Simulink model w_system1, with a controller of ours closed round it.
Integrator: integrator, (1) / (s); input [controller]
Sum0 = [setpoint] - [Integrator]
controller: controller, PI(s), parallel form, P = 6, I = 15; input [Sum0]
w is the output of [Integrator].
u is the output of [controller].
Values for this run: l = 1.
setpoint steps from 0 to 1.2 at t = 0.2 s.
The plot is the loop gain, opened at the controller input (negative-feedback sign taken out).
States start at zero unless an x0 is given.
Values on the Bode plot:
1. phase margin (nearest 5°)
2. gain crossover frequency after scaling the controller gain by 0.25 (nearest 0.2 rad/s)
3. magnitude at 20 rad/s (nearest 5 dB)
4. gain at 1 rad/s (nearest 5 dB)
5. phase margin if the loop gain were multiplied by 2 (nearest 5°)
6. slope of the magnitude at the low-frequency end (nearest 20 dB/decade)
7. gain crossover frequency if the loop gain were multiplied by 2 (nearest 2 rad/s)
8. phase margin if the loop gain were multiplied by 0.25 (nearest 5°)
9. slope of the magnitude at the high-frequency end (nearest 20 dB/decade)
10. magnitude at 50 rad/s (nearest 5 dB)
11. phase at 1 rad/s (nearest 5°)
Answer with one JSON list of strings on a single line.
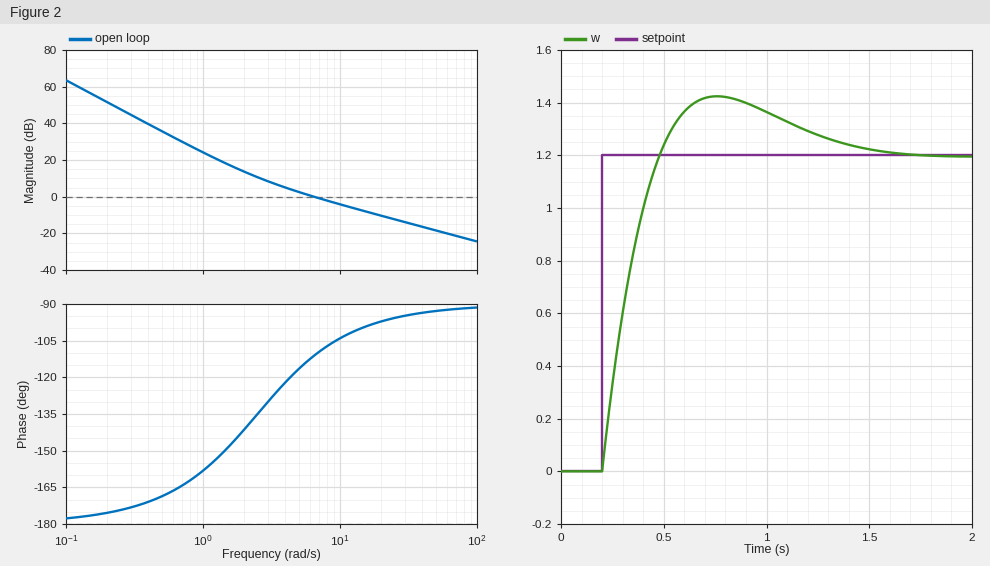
["70°", "2.2 rad/s", "-10 dB", "25 dB", "80°", "-40 dB/decade", "12 rad/s", "40°", "-20 dB/decade", "-20 dB", "-160°"]
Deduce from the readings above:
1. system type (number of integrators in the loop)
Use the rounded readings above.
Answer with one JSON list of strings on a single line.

["2"]
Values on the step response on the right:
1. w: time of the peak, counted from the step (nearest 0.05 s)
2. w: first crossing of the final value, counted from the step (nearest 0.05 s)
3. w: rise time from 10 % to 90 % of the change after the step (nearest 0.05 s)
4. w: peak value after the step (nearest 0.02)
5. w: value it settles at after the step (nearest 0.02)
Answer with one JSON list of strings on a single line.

["0.55 s", "0.30 s", "0.20 s", "1.42", "1.20"]
